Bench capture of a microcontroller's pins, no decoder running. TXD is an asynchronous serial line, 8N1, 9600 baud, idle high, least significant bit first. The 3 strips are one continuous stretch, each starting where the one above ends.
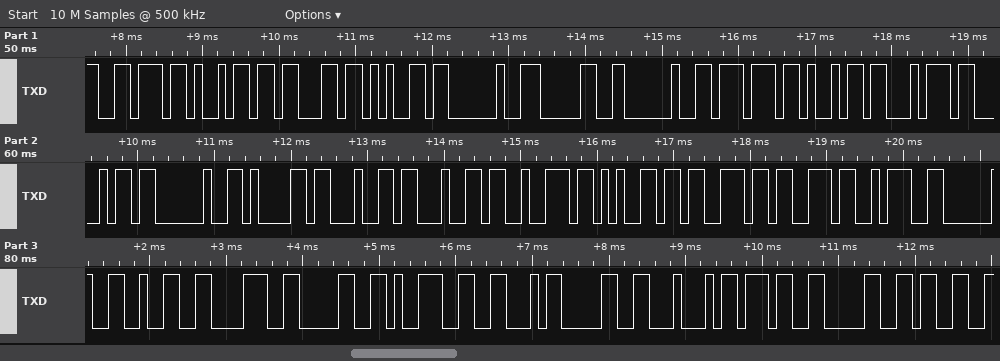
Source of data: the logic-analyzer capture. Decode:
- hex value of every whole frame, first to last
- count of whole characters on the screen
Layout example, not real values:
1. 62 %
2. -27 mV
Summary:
1. 76 69 63 65 20 30 20 77 69 74 68 20 61 64 64 72 65 73 73 3A 20 32 38 30 39 46 30 44 37 30 33
2. 31
